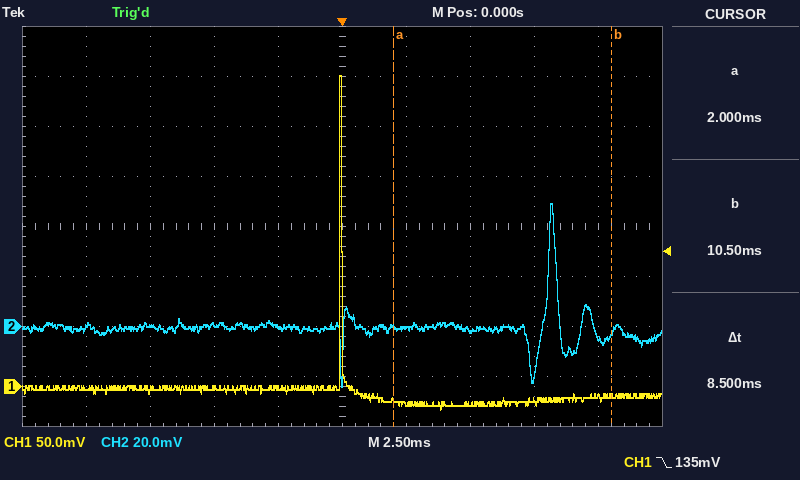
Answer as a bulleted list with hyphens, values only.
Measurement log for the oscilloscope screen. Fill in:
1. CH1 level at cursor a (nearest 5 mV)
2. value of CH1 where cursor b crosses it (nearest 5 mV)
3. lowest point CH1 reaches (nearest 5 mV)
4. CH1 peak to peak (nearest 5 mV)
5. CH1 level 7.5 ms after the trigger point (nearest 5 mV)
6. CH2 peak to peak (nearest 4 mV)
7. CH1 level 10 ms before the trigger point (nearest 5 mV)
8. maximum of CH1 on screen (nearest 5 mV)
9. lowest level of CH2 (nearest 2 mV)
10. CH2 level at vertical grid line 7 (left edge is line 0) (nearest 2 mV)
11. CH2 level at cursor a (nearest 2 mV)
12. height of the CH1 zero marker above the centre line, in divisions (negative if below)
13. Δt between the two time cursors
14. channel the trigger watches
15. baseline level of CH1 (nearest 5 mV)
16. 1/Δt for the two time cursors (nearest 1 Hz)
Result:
- -15 mV
- -10 mV
- -25 mV
- 335 mV
- -15 mV
- 72 mV
- 0 mV
- 310 mV
- -24 mV
- -2 mV
- 0 mV
- -3.2 div
- 8.5 ms
- CH1
- 0 mV
- 118 Hz
